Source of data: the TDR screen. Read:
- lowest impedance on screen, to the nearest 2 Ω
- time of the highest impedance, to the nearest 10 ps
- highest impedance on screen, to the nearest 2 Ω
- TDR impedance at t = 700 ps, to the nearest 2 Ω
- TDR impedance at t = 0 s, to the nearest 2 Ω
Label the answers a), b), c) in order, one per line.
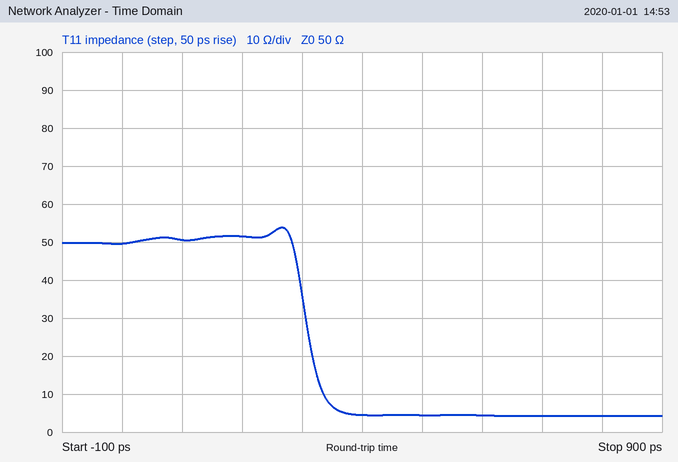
a) 4 Ω
b) 270 ps
c) 54 Ω
d) 4 Ω
e) 50 Ω
